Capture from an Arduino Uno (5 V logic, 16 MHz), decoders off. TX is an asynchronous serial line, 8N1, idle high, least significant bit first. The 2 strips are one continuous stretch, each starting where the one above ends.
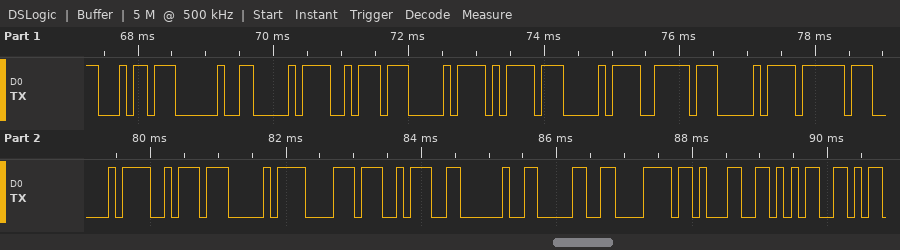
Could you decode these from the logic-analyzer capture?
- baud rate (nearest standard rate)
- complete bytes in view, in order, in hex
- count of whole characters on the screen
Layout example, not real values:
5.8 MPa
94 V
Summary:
9600 baud
0xB4 0x20 0xD0 0xBA 0xD0 0xBD 0xD0 0xBE 0xD0 0xBF 0xD0 0xBA 0xD0 0xB8 0x3A 0x20 0x30 0x78 0x31 0x35
20
